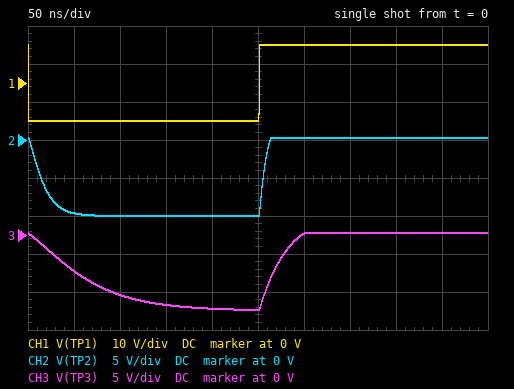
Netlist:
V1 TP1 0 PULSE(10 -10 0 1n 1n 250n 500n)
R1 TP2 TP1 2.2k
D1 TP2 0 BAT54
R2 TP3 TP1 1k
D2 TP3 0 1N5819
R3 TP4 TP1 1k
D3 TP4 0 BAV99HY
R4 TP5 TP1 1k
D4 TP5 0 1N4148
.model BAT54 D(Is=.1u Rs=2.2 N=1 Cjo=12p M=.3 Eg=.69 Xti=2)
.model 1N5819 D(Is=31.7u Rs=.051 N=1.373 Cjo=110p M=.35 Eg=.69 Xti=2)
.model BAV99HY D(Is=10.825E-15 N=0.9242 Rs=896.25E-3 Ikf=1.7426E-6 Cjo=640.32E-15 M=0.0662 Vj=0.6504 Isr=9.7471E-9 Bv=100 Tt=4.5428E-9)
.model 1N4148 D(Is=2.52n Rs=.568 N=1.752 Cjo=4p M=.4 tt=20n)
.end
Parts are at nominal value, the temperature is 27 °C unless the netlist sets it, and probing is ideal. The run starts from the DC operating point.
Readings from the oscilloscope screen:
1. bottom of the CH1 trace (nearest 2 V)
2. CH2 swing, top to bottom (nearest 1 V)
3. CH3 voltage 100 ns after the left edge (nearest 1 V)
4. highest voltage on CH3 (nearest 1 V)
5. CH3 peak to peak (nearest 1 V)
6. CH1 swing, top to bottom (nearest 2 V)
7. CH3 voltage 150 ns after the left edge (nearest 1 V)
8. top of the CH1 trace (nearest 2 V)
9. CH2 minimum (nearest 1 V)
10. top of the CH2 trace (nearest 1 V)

-10 V
10 V
-8 V
0 V
10 V
20 V
-9 V
10 V
-10 V
0 V
